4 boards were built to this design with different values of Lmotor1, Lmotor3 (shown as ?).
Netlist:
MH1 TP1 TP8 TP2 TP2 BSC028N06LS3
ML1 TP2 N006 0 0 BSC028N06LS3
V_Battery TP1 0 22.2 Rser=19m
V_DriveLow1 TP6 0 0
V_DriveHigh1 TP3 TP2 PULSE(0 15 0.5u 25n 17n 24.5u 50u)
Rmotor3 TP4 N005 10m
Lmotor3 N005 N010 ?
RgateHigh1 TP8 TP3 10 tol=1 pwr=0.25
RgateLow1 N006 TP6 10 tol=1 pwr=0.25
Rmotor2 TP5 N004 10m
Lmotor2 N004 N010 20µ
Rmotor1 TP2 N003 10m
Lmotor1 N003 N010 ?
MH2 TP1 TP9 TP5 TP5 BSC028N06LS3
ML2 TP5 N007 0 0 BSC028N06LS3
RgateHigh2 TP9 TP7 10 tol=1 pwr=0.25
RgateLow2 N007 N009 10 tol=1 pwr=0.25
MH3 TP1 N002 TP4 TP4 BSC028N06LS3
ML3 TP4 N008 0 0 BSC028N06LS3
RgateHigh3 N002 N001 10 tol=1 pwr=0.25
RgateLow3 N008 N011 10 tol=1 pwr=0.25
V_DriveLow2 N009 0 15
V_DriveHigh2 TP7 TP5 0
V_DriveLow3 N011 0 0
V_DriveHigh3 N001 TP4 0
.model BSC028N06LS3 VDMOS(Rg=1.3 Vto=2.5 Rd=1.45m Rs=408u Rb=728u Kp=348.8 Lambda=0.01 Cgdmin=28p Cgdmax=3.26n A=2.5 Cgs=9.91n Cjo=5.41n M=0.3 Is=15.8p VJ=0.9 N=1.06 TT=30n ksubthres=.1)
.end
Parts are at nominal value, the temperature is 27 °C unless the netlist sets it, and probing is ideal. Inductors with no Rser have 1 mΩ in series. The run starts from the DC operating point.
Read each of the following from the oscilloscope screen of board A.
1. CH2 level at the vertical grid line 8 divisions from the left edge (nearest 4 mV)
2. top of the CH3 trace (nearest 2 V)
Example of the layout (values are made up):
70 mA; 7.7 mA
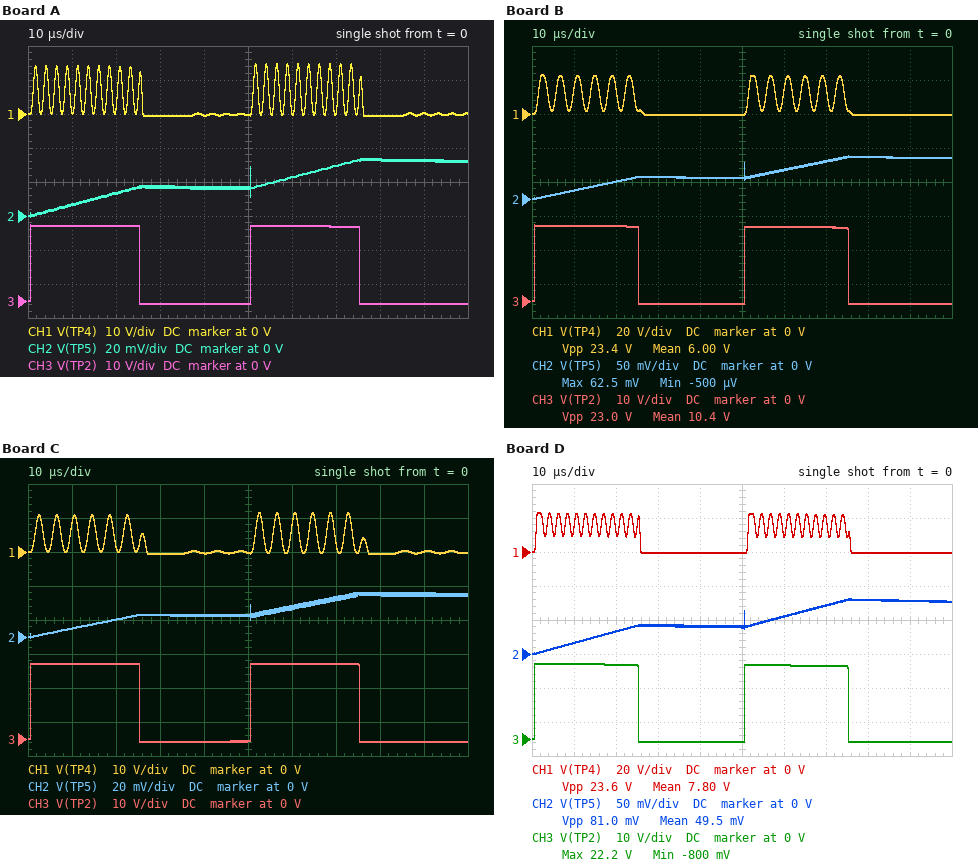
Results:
32 mV; 22 V
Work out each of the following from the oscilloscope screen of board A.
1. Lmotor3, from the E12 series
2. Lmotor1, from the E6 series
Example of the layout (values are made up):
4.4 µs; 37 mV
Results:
12 µH; 47 µH
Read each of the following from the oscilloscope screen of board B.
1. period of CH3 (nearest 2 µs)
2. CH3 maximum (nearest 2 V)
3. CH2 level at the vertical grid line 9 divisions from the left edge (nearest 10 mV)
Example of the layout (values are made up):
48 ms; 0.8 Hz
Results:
50 µs; 22 V; 60 mV
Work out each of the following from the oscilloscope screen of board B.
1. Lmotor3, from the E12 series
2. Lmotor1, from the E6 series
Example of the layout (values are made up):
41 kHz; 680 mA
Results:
68 µH; 15 µH
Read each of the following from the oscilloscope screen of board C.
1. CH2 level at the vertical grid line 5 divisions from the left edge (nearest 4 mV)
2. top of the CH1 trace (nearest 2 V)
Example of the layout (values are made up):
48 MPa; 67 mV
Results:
12 mV; 12 V
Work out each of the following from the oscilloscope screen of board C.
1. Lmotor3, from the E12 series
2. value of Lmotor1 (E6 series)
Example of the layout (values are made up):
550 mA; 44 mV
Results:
56 µH; 68 µH
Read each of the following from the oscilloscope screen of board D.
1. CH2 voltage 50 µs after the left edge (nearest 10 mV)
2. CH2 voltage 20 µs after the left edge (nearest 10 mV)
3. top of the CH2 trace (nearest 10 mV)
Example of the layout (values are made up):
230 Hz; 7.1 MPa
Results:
40 mV; 30 mV; 80 mV
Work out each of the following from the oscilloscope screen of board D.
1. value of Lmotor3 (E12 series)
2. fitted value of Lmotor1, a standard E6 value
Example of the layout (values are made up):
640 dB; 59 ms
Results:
15 µH; 6.8 µH
